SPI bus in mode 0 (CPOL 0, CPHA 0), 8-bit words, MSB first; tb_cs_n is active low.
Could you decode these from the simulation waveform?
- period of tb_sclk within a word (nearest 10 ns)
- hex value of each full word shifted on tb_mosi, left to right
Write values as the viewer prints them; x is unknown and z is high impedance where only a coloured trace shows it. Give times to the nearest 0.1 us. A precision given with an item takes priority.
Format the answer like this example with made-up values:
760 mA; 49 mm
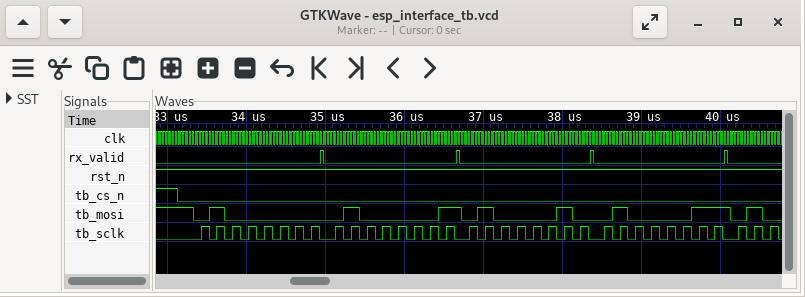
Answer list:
200 ns; 40, 41, 42, 43
